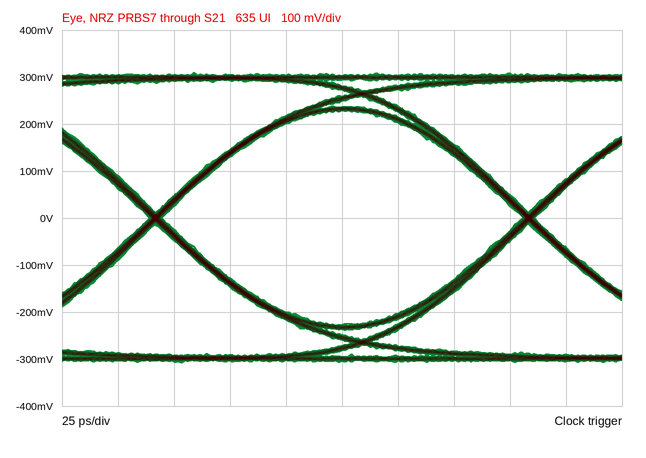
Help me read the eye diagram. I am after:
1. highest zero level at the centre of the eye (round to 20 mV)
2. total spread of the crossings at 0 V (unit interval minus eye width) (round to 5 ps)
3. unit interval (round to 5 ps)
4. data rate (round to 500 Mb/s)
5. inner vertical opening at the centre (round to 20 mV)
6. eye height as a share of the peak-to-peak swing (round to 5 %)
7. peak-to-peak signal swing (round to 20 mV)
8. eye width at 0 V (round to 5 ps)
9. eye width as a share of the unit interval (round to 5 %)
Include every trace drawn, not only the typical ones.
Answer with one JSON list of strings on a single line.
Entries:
["-220 mV", "5 ps", "165 ps", "6.0 Gb/s", "460 mV", "75 %", "620 mV", "160 ps", "95 %"]
